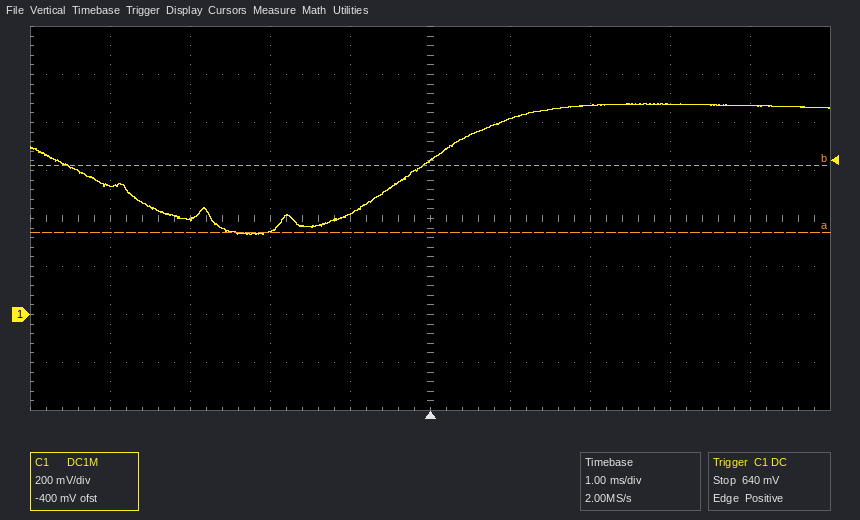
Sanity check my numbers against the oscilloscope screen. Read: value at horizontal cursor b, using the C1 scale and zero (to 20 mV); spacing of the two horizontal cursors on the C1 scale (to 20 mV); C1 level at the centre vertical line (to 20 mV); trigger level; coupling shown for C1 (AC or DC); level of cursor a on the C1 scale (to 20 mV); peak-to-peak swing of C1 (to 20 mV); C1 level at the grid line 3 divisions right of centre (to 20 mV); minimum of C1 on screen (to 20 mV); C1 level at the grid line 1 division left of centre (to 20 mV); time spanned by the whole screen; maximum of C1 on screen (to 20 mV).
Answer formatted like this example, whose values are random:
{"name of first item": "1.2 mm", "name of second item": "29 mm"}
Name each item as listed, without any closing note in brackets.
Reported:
{"value at horizontal cursor b, using the C1 scale and zero": "620 mV", "spacing of the two horizontal cursors on the C1 scale": "280 mV", "C1 level at the centre vertical line": "640 mV", "trigger level": "640 mV", "coupling shown for C1": "DC", "level of cursor a on the C1 scale": "340 mV", "peak-to-peak swing of C1": "540 mV", "C1 level at the grid line 3 divisions right of centre": "880 mV", "minimum of C1 on screen": "340 mV", "C1 level at the grid line 1 division left of centre": "420 mV", "time spanned by the whole screen": "10 ms", "maximum of C1 on screen": "880 mV"}
